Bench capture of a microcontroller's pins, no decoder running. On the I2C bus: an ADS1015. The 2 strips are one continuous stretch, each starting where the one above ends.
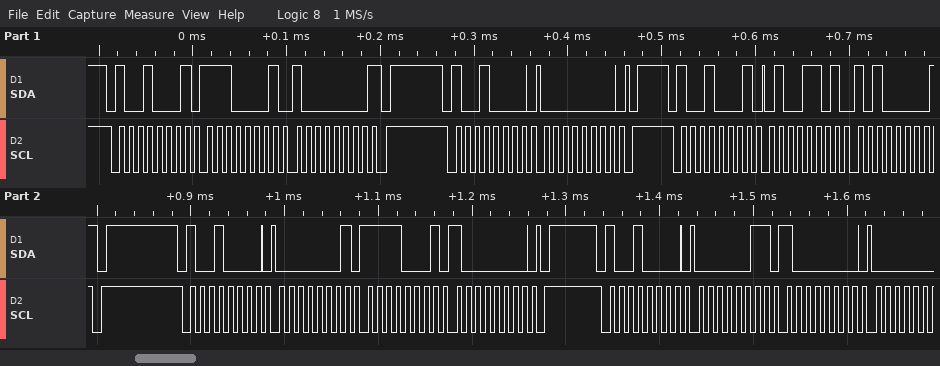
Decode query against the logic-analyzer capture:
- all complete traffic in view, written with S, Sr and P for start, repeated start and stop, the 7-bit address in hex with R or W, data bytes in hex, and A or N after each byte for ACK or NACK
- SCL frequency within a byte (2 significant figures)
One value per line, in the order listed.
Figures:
S 48R A E1 A 80 N P S 48W A 00 A P S 48R A 4D A A0 N P S 48W A 01 A F1 A 80 A P S 48W A 03 A 80 A
100 kHz
